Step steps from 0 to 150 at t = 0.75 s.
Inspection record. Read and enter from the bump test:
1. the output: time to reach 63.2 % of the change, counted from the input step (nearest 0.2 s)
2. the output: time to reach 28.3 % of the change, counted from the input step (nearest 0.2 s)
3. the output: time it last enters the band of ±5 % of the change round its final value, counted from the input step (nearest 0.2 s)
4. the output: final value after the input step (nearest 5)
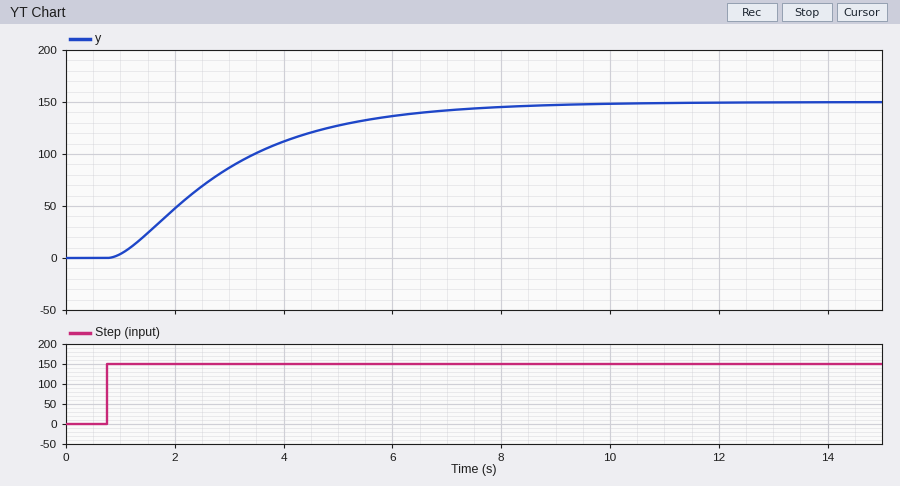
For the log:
2.6 s
1.2 s
6.4 s
150
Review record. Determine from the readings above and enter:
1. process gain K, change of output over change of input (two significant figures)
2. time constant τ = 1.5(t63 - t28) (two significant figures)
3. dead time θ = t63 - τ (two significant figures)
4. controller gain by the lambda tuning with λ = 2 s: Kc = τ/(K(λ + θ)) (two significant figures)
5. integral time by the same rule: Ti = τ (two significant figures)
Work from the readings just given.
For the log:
1.0
2.1 s
0.50 s
0.84
2.1 s
